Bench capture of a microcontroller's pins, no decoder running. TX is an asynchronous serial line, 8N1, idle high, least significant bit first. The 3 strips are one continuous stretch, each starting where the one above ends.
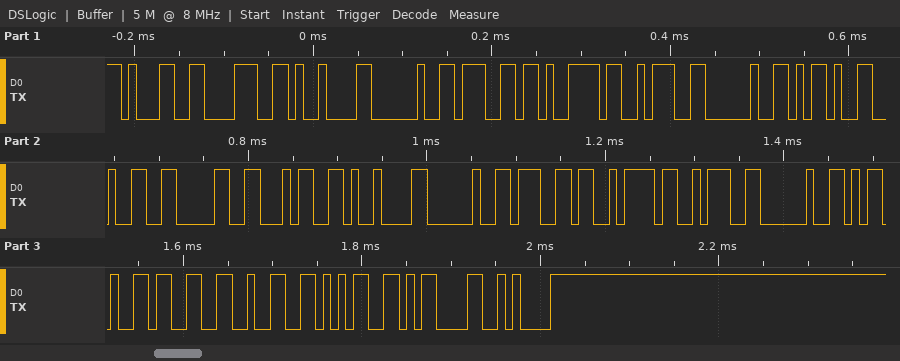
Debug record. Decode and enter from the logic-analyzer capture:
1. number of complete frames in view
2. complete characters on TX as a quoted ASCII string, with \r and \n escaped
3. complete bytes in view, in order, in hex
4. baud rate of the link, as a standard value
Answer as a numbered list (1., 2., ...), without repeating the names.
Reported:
1. 24
2. "18\t gy: -204\t gz: -325\r\n"
3. 31 38 09 20 67 79 3A 20 2D 32 30 34 09 20 67 7A 3A 20 2D 33 32 35 0D 0A
4. 115200 baud
